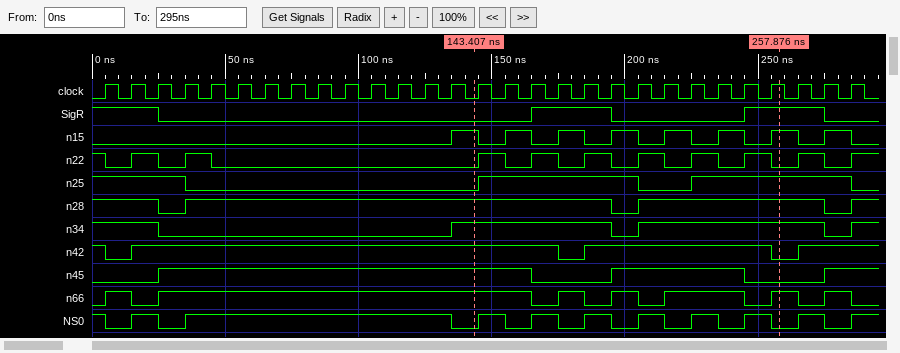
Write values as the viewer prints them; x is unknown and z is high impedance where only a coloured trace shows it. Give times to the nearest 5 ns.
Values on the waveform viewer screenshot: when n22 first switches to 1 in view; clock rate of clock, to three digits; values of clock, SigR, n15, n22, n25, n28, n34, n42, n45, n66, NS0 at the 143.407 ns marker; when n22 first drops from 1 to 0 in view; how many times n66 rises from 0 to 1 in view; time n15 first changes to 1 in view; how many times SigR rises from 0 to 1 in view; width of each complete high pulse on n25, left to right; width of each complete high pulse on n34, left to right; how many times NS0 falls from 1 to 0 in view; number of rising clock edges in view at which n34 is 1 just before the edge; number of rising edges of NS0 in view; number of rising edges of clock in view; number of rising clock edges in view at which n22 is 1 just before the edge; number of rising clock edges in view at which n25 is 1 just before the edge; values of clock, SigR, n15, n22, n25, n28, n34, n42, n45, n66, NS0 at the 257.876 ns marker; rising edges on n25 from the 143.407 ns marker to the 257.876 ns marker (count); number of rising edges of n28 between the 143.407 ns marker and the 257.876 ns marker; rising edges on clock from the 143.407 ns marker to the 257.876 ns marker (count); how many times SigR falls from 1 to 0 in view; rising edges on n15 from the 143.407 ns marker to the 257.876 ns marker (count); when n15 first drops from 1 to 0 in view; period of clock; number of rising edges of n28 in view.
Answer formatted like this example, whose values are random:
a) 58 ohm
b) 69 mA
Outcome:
a) 15 ns
b) 100 MHz
c) clock=0, SigR=0, n15=1, n22=0, n25=0, n28=1, n34=1, n42=1, n45=1, n66=1, NS0=0
d) 5 ns
e) 7
f) 135 ns
g) 2
h) 60 ns, 60 ns
i) 60 ns, 70 ns
j) 10
k) 16
l) 10
m) 29
n) 10
o) 16
p) clock=1, SigR=1, n15=1, n22=0, n25=1, n28=1, n34=1, n42=0, n45=0, n66=1, NS0=0
q) 2
r) 1
s) 12
t) 3
u) 6
v) 145 ns
w) 10 ns
x) 3
